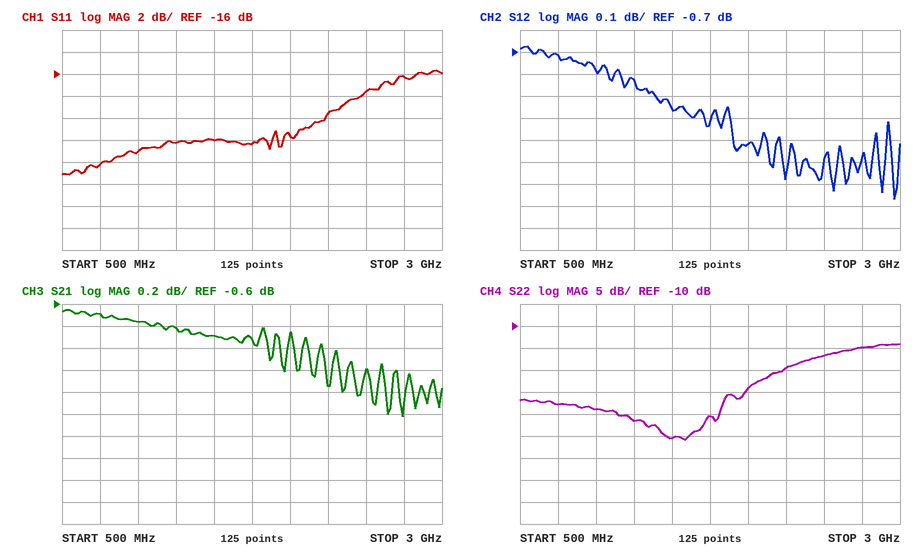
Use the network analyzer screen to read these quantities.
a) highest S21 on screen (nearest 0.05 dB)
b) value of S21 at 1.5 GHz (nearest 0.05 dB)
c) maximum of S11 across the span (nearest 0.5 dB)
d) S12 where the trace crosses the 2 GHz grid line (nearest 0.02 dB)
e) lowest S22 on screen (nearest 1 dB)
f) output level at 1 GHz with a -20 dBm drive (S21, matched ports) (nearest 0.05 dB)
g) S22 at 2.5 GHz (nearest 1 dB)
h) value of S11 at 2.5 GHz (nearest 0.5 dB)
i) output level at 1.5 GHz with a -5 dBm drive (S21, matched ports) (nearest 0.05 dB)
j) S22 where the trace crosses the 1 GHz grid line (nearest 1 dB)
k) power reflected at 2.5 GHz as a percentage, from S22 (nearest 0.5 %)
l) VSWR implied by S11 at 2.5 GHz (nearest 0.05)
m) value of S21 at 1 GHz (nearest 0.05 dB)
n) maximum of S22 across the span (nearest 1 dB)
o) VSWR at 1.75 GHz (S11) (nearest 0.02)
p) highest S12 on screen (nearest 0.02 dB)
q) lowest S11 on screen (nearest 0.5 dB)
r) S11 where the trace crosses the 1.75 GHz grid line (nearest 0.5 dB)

-0.65 dB
-0.90 dB
-15.5 dB
-1.12 dB
-36 dB
-20.75 dBm
-17 dB
-17.5 dB
-5.90 dBm
-29 dB
2.0 %
1.30
-0.75 dB
-14 dB
1.16
-0.68 dB
-25.0 dB
-22.5 dB
